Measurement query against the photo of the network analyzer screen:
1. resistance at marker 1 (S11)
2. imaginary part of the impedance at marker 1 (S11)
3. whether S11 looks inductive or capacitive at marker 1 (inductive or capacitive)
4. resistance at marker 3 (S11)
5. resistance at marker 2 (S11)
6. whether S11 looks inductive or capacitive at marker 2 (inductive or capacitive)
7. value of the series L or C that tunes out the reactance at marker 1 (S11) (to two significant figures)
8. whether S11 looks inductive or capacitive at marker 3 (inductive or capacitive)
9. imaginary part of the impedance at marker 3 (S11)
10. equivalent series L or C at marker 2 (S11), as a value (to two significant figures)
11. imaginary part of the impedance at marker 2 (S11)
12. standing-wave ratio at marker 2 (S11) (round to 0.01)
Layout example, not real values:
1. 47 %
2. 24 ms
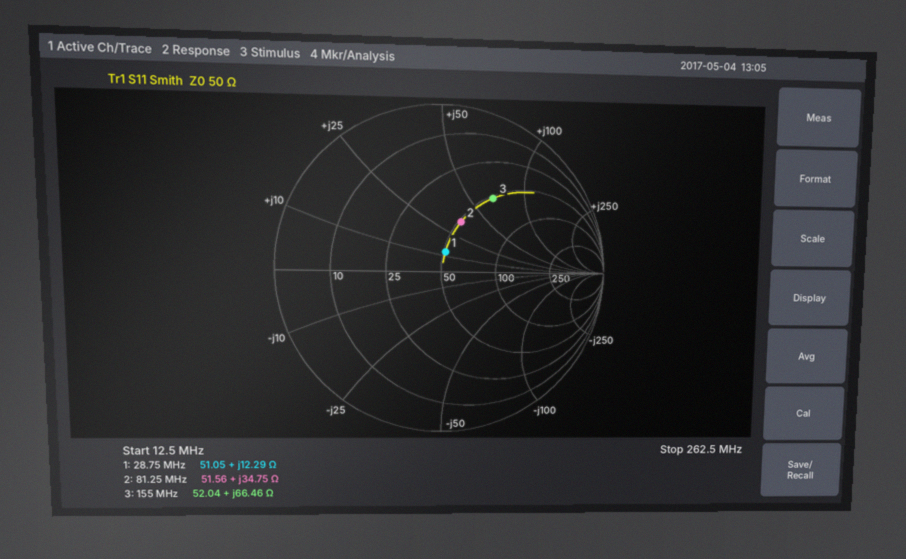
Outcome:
1. 51.05 Ω
2. +12.29 Ω
3. inductive
4. 52.04 Ω
5. 51.56 Ω
6. inductive
7. 450 pF
8. inductive
9. +66.46 Ω
10. 68 nH
11. +34.75 Ω
12. 1.96
